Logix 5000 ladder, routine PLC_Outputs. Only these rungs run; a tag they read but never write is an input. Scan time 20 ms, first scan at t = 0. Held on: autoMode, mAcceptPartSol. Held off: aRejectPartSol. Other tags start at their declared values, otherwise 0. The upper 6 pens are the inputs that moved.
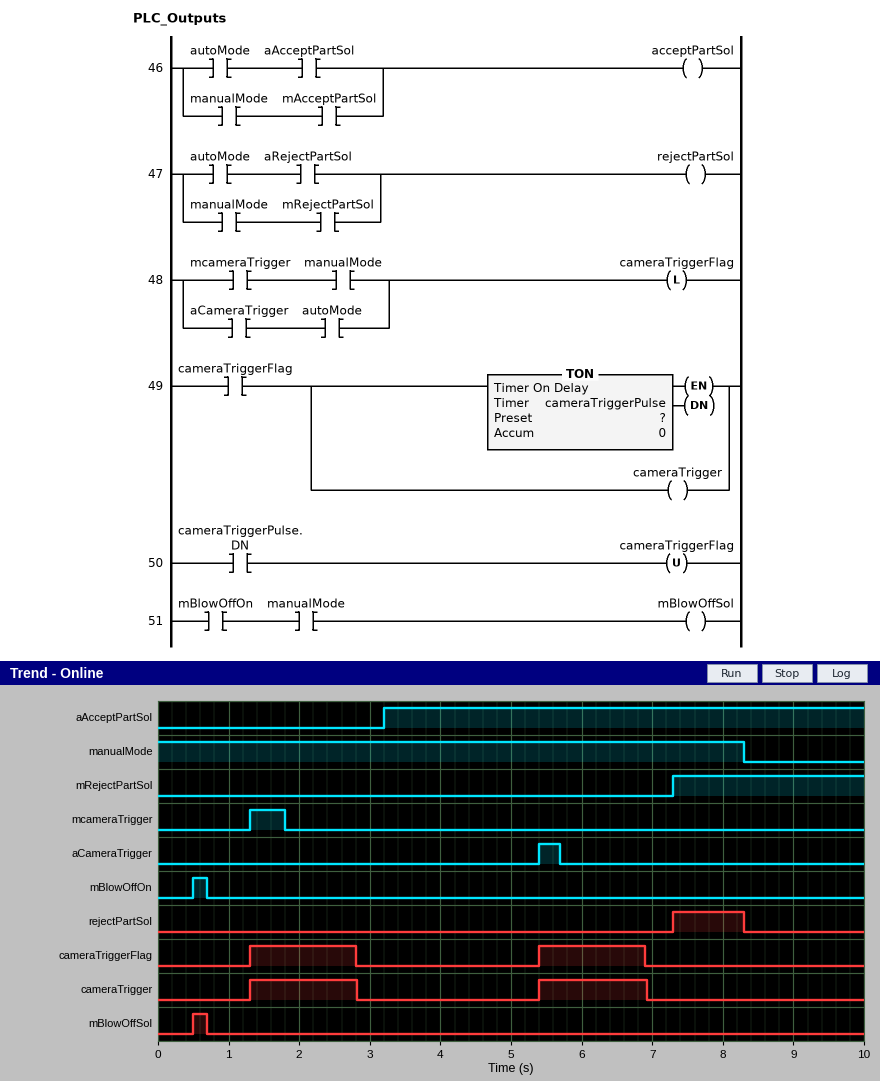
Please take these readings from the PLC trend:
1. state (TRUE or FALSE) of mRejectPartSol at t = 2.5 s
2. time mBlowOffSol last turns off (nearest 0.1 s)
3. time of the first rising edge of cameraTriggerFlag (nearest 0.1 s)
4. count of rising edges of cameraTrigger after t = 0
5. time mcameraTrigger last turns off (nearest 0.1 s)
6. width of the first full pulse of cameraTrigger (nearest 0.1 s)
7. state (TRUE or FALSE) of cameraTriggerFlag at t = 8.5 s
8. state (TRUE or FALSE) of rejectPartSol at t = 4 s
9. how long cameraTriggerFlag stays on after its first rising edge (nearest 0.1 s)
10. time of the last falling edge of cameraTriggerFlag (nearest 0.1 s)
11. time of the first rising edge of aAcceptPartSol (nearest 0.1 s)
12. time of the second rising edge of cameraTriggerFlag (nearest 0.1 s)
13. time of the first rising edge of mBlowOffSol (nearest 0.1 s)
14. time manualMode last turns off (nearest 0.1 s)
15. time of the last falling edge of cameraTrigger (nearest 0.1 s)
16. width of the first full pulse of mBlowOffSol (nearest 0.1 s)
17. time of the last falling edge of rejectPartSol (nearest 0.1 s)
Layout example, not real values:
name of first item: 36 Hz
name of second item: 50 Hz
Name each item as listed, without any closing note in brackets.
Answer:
state (TRUE or FALSE) of mRejectPartSol at t = 2.5 s: FALSE
time mBlowOffSol last turns off: 0.7 s
time of the first rising edge of cameraTriggerFlag: 1.3 s
count of rising edges of cameraTrigger after t = 0: 2
time mcameraTrigger last turns off: 1.8 s
width of the first full pulse of cameraTrigger: 1.5 s
state (TRUE or FALSE) of cameraTriggerFlag at t = 8.5 s: FALSE
state (TRUE or FALSE) of rejectPartSol at t = 4 s: FALSE
how long cameraTriggerFlag stays on after its first rising edge: 1.5 s
time of the last falling edge of cameraTriggerFlag: 6.9 s
time of the first rising edge of aAcceptPartSol: 3.2 s
time of the second rising edge of cameraTriggerFlag: 5.4 s
time of the first rising edge of mBlowOffSol: 0.5 s
time manualMode last turns off: 8.3 s
time of the last falling edge of cameraTrigger: 6.9 s
width of the first full pulse of mBlowOffSol: 0.2 s
time of the last falling edge of rejectPartSol: 8.3 s
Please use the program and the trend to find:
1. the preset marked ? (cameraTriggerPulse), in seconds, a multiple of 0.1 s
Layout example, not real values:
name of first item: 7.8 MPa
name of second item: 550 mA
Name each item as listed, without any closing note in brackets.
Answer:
the preset marked ? (cameraTriggerPulse), in seconds, a multiple of 0.1 s: 1.5 s
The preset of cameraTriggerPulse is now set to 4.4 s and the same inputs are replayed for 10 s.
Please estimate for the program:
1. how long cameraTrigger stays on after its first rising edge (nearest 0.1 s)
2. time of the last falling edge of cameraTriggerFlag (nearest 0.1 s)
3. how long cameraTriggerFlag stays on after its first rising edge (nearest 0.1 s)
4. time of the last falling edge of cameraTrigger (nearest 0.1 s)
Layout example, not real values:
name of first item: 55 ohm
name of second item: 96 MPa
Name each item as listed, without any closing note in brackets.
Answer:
how long cameraTrigger stays on after its first rising edge: 4.4 s
time of the last falling edge of cameraTriggerFlag: 5.7 s
how long cameraTriggerFlag stays on after its first rising edge: 4.4 s
time of the last falling edge of cameraTrigger: 5.7 s
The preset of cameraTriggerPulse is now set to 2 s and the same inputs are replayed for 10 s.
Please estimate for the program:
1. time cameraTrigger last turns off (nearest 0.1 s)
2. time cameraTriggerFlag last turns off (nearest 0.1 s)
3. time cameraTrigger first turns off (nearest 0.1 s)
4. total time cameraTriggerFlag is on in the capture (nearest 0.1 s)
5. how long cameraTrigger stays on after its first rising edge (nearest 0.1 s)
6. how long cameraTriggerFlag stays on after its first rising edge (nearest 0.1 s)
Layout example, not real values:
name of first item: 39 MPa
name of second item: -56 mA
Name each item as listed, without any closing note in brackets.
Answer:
time cameraTrigger last turns off: 7.4 s
time cameraTriggerFlag last turns off: 7.4 s
time cameraTrigger first turns off: 3.3 s
total time cameraTriggerFlag is on in the capture: 4.0 s
how long cameraTrigger stays on after its first rising edge: 2.0 s
how long cameraTriggerFlag stays on after its first rising edge: 2.0 s
